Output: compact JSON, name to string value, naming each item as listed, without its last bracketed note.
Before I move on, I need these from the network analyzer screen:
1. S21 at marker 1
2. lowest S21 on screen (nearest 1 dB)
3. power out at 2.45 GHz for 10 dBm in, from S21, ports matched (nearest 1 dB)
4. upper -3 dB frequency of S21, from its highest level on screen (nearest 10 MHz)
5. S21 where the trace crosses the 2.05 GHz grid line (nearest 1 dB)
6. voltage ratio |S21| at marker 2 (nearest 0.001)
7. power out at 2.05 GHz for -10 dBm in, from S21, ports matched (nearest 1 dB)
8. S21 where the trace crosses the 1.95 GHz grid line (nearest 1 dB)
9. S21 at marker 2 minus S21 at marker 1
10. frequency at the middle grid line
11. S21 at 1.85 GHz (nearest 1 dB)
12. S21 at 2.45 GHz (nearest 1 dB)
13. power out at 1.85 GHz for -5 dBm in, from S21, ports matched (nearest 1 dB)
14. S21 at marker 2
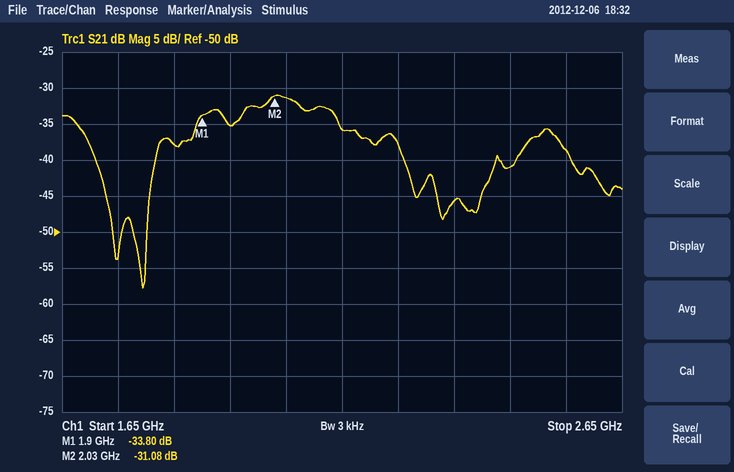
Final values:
{"S21 at marker 1": "-33.80 dB", "lowest S21 on screen": "-58 dB", "power out at 2.45 GHz for 10 dBm in, from S21, ports matched": "-31 dBm", "upper -3 dB frequency of S21, from its highest level on screen": "2.14 GHz", "S21 where the trace crosses the 2.05 GHz grid line": "-31 dB", "voltage ratio |S21| at marker 2": "0.028", "power out at 2.05 GHz for -10 dBm in, from S21, ports matched": "-41 dBm", "S21 where the trace crosses the 1.95 GHz grid line": "-35 dB", "S21 at marker 2 minus S21 at marker 1": "2.72 dB", "frequency at the middle grid line": "2.15 GHz", "S21 at 1.85 GHz": "-38 dB", "S21 at 2.45 GHz": "-41 dB", "power out at 1.85 GHz for -5 dBm in, from S21, ports matched": "-43 dBm", "S21 at marker 2": "-31.08 dB"}
